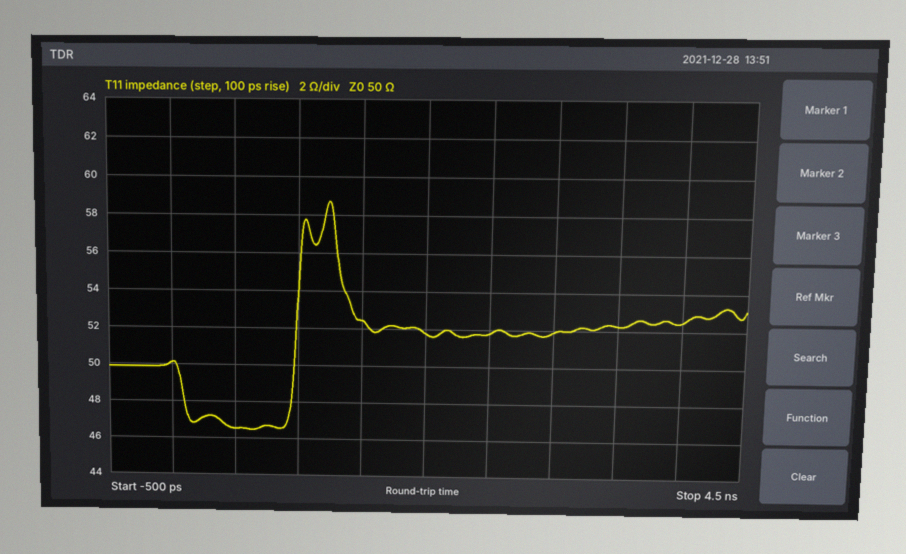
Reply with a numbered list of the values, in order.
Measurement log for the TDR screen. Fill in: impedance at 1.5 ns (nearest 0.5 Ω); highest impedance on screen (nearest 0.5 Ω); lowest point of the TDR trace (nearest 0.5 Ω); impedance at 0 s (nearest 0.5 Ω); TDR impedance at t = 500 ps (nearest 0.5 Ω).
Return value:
1. 52.5 Ω
2. 58.5 Ω
3. 46.5 Ω
4. 50.0 Ω
5. 46.5 Ω
